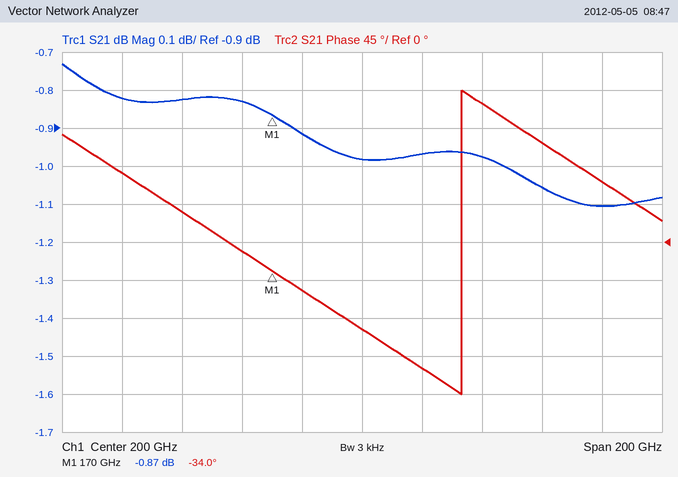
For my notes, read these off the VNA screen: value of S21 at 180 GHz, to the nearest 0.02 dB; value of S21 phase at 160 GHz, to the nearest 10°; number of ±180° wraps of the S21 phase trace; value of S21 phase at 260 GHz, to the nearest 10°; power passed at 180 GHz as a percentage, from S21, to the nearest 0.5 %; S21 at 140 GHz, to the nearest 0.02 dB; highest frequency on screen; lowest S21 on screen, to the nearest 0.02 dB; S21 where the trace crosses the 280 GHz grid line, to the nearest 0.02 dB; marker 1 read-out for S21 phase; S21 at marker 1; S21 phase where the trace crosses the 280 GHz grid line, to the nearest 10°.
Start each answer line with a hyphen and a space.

- -0.92 dB
- -10°
- 1
- 120°
- 81.0 %
- -0.82 dB
- 300 GHz
- -1.10 dB
- -1.10 dB
- -34.0°
- -0.87 dB
- 70°
